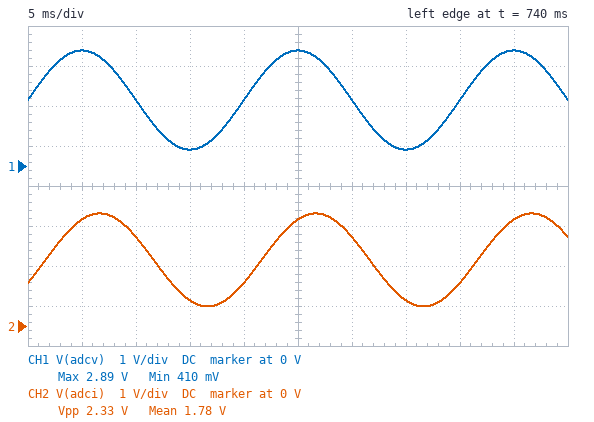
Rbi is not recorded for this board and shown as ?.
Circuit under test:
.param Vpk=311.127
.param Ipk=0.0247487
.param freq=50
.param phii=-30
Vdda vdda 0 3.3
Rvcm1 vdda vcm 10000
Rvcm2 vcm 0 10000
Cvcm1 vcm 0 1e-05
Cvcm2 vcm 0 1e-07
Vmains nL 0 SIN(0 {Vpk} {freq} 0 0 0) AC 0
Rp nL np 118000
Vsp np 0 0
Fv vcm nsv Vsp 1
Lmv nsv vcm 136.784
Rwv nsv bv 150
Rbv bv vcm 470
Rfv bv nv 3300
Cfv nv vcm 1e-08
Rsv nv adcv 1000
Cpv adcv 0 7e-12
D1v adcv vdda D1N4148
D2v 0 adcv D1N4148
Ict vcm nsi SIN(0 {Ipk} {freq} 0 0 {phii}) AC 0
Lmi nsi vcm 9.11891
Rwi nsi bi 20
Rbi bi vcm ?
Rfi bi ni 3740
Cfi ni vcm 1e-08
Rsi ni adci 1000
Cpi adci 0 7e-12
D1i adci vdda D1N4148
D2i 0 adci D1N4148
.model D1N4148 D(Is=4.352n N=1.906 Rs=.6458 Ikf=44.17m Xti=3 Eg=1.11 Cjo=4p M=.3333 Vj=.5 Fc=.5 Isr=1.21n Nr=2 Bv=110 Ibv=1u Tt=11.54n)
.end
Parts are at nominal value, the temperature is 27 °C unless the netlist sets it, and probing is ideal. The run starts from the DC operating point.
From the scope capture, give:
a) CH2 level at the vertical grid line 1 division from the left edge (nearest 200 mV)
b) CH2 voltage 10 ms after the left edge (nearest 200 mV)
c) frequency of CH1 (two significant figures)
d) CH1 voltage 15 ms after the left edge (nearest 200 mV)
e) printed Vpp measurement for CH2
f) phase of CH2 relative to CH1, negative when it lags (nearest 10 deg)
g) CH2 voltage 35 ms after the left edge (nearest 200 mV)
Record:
2.6 V
2.2 V
50 Hz
400 mV
2.33 V
-30 deg
600 mV
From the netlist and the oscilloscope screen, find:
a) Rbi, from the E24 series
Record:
47 Ω
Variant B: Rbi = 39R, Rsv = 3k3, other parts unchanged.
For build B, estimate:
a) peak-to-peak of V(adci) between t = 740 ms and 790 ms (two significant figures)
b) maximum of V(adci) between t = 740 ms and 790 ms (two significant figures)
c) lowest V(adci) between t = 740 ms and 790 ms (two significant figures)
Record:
1.9 V
2.6 V
690 mV
